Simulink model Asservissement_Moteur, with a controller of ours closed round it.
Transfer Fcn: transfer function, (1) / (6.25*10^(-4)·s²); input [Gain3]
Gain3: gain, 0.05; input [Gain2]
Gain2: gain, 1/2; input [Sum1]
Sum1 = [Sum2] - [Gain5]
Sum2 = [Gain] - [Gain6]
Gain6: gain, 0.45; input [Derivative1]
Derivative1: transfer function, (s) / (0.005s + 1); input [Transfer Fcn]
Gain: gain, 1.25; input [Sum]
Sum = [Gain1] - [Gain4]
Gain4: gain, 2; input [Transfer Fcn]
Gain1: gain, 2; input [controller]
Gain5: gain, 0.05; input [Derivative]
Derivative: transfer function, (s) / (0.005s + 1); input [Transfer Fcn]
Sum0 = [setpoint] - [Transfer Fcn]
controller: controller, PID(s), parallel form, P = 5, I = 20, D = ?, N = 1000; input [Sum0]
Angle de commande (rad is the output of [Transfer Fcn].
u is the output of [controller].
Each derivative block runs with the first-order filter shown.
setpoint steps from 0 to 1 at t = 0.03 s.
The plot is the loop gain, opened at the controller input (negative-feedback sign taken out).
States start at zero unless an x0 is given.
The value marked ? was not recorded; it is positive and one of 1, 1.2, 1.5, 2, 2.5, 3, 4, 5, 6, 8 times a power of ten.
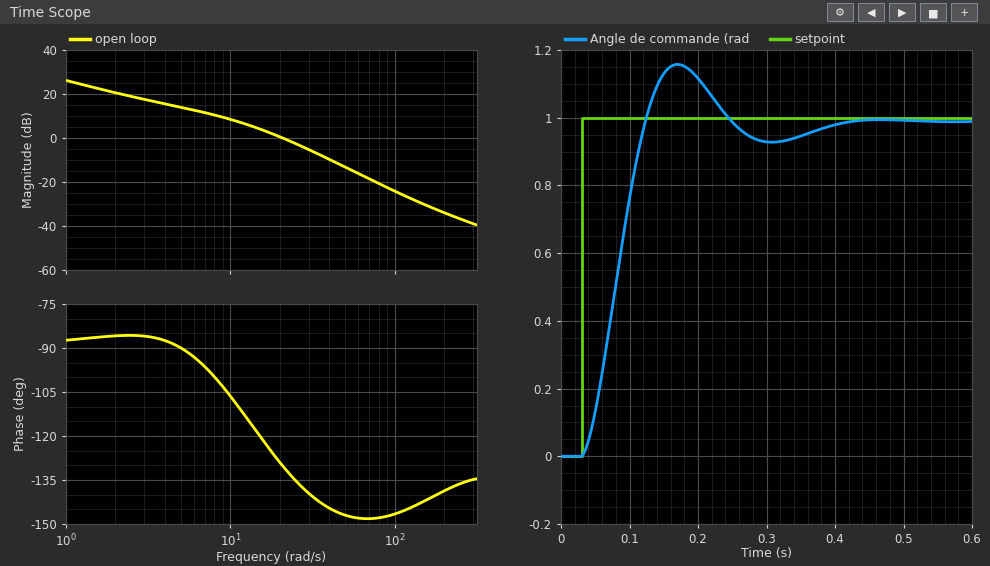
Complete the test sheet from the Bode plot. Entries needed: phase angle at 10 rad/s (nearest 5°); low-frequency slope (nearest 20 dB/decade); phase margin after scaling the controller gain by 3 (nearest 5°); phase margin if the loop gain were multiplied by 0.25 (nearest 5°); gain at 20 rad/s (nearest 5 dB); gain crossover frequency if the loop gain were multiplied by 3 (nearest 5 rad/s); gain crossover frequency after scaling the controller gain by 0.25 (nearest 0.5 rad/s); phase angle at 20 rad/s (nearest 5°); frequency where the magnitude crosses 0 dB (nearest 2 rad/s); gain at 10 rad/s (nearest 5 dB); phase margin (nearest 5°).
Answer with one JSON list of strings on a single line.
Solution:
["-105°", "-20 dB/decade", "35°", "85°", "0 dB", "40 rad/s", "6.5 rad/s", "-130°", "20 rad/s", "10 dB", "50°"]
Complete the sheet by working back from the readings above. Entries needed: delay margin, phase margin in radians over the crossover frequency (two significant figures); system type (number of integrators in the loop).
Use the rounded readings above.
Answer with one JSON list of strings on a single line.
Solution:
["0.044 s", "1"]
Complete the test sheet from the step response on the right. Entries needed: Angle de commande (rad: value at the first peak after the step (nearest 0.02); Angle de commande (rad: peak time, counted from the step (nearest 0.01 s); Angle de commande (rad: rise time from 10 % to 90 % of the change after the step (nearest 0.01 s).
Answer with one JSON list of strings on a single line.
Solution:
["1.16", "0.14 s", "0.07 s"]
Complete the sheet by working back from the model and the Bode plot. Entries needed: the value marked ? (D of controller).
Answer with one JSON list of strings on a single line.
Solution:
["0.025"]
